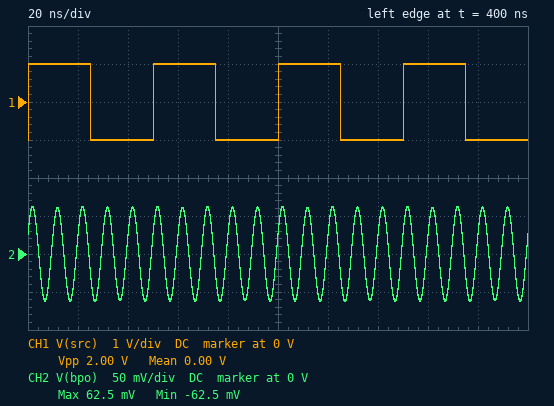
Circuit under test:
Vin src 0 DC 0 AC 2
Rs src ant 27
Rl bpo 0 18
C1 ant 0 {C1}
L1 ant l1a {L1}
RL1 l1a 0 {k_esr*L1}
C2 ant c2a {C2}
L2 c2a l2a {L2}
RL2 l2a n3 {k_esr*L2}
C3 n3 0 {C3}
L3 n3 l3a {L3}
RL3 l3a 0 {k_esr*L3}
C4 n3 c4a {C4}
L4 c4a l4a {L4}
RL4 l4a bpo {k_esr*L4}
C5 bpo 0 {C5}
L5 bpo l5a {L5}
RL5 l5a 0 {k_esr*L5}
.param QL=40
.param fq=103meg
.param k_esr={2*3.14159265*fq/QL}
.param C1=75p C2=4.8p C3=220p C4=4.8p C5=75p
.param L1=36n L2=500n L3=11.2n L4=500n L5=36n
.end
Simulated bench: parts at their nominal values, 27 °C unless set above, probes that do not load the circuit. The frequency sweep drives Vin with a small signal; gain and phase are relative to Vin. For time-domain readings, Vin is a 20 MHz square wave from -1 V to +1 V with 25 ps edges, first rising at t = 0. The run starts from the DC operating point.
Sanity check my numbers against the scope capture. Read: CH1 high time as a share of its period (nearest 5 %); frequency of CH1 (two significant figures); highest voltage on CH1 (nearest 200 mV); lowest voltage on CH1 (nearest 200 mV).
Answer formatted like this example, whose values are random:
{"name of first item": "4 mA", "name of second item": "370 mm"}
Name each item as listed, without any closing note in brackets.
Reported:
{"CH1 high time as a share of its period": "50 %", "frequency of CH1": "20 MHz", "highest voltage on CH1": "1.0 V", "lowest voltage on CH1": "-1.0 V"}
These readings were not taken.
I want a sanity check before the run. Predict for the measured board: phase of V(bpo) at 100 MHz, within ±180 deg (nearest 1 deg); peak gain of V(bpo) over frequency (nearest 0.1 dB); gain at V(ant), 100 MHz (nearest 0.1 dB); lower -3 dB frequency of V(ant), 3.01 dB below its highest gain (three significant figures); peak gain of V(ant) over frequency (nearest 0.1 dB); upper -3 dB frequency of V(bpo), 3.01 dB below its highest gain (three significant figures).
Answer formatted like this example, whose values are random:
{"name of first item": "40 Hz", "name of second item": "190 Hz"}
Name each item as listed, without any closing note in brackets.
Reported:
{"phase of V(bpo) at 100 MHz, within ±180 deg": "30 deg", "peak gain of V(bpo) over frequency": "-11.3 dB", "gain at V(ant), 100 MHz": "-3.7 dB", "lower -3 dB frequency of V(ant), 3.01 dB below its highest gain": "61.7 MHz", "peak gain of V(ant) over frequency": "-0.6 dB", "upper -3 dB frequency of V(bpo), 3.01 dB below its highest gain": "115 MHz"}
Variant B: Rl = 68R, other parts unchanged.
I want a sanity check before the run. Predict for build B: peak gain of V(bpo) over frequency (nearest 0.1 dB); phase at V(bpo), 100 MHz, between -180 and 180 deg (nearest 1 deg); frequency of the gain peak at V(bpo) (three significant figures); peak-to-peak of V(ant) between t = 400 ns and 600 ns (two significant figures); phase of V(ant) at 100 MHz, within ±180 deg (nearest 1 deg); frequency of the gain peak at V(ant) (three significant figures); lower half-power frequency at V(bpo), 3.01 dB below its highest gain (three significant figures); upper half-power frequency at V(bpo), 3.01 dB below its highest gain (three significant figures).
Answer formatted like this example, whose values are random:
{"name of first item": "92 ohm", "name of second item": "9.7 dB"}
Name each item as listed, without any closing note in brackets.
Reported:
{"peak gain of V(bpo) over frequency": "-5.0 dB", "phase at V(bpo), 100 MHz, between -180 and 180 deg": "17 deg", "frequency of the gain peak at V(bpo)": "107 MHz", "peak-to-peak of V(ant) between t = 400 ns and 600 ns": "1.8 V", "phase of V(ant) at 100 MHz, within ±180 deg": "-8 deg", "frequency of the gain peak at V(ant)": "83.9 MHz", "lower half-power frequency at V(bpo), 3.01 dB below its highest gain": "91.4 MHz", "upper half-power frequency at V(bpo), 3.01 dB below its highest gain": "116 MHz"}
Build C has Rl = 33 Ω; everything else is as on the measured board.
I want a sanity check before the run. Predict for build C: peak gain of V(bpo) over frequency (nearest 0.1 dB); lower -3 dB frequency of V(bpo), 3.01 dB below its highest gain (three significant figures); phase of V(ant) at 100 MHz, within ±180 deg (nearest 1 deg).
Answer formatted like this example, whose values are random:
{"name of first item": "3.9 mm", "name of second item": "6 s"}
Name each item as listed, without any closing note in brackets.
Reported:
{"peak gain of V(bpo) over frequency": "-8.2 dB", "lower -3 dB frequency of V(bpo), 3.01 dB below its highest gain": "91.5 MHz", "phase of V(ant) at 100 MHz, within ±180 deg": "-13 deg"}
